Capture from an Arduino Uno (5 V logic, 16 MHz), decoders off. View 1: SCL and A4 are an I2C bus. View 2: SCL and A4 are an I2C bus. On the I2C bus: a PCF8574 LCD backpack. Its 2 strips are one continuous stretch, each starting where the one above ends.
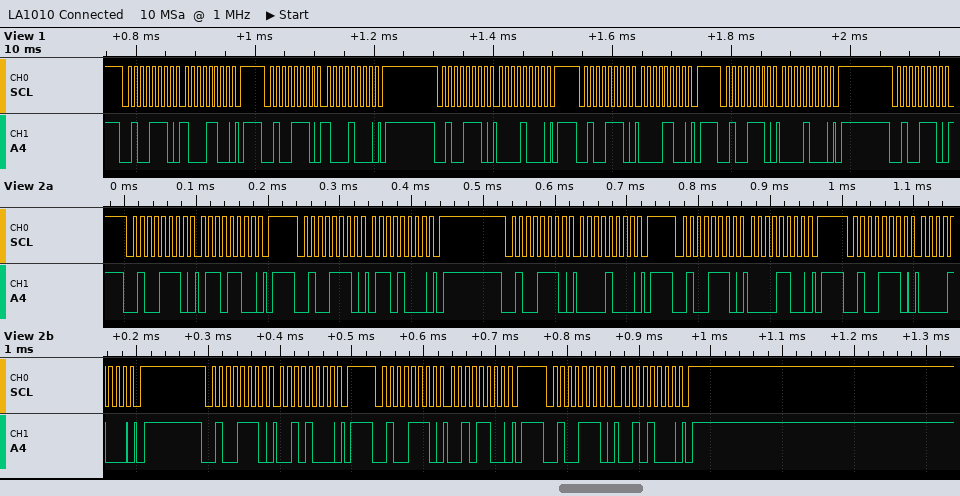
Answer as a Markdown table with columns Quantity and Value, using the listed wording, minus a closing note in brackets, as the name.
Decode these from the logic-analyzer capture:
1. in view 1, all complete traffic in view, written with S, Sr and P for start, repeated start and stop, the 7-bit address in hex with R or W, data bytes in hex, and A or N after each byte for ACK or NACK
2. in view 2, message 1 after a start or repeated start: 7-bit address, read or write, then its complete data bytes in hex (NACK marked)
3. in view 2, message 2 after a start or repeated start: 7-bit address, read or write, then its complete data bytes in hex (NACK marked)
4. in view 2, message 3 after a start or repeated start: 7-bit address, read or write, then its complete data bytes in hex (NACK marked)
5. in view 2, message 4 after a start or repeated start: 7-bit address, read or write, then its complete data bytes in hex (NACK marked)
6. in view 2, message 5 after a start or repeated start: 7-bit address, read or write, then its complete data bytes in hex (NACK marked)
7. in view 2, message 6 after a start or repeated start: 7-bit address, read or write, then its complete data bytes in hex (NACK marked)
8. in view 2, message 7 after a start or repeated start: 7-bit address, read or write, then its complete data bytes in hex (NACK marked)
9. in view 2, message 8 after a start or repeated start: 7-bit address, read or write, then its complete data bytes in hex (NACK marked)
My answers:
| Quantity | Value |
|---|---|
| in view 1, all complete traffic in view, written with S, Sr and P for start, repeated start and stop, the 7-bit address in hex with R or W, data bytes in hex, and A or N after each byte for ACK or NACK | S 27W A 8C A P S 27W A 88 A P S 27W A 08 A P S 27W A 0C A P S 27W A 08 A P S 27W A |
| in view 2, message 1 after a start or repeated start: 7-bit address, read or write, then its complete data bytes in hex | 0x27 write: 6C |
| in view 2, message 2 after a start or repeated start: 7-bit address, read or write, then its complete data bytes in hex | 0x27 write: 68 |
| in view 2, message 3 after a start or repeated start: 7-bit address, read or write, then its complete data bytes in hex | 0x27 write: 08 |
| in view 2, message 4 after a start or repeated start: 7-bit address, read or write, then its complete data bytes in hex | 0x27 write: 0C |
| in view 2, message 5 after a start or repeated start: 7-bit address, read or write, then its complete data bytes in hex | 0x27 write: 08 |
| in view 2, message 6 after a start or repeated start: 7-bit address, read or write, then its complete data bytes in hex | 0x27 write: 28 |
| in view 2, message 7 after a start or repeated start: 7-bit address, read or write, then its complete data bytes in hex | 0x27 write: 2C |
| in view 2, message 8 after a start or repeated start: 7-bit address, read or write, then its complete data bytes in hex | 0x27 write: 28 |
